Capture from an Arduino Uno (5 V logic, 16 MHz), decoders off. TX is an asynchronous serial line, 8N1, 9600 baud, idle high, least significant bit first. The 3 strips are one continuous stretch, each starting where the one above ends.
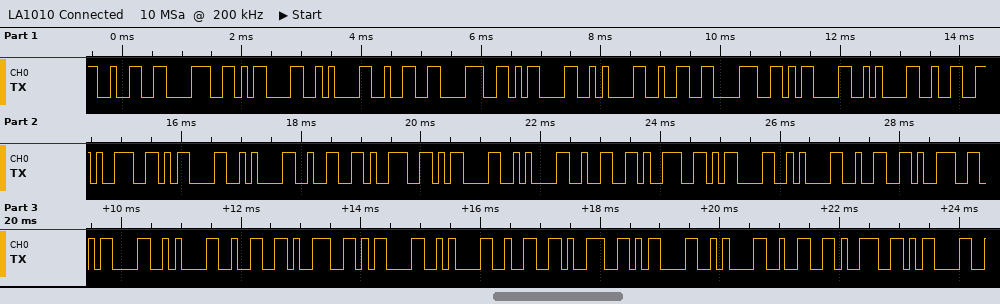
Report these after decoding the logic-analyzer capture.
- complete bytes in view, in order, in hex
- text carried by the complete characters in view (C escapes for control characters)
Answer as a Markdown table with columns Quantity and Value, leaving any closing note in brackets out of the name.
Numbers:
| Quantity | Value |
|---|---|
| complete bytes in view, in order, in hex | 0x32 0x38 0x0D 0x0A 0x32 0x38 0x0D 0x0A 0x32 0x38 0x0D 0x0A 0x32 0x39 0x0D 0x0A 0x32 0x39 0x0D 0x0A 0x32 0x39 0x0D 0x0A 0x32 0x39 0x0D 0x0A 0x32 0x39 0x0D 0x0A 0x32 0x39 0x0D 0x0A 0x32 0x39 0x0D |
| text carried by the complete characters in view | "28\r\n28\r\n28\r\n29\r\n29\r\n29\r\n29\r\n29\r\n29\r\n29\r" |
